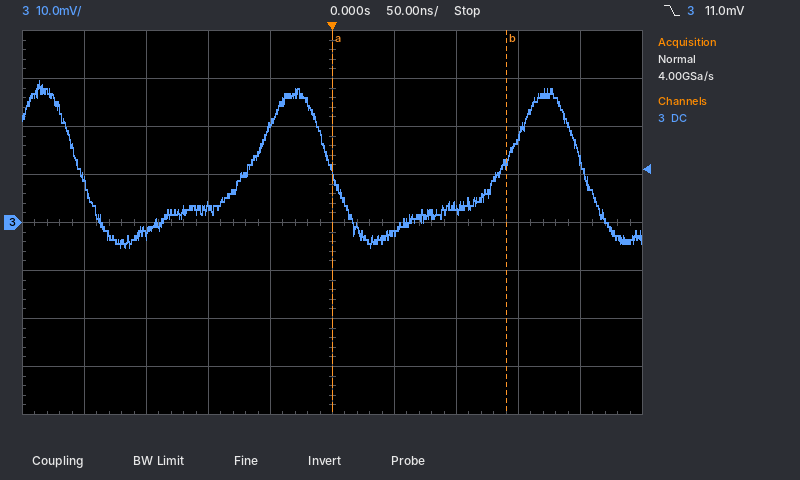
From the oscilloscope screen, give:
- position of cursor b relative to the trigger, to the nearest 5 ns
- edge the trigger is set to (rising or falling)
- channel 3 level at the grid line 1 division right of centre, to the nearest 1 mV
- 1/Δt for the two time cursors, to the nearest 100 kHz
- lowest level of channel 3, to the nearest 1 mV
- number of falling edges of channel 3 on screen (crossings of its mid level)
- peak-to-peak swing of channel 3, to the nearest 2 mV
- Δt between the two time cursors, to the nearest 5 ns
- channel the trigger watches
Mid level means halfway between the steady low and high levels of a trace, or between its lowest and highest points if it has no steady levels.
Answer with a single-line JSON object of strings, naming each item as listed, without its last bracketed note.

{"position of cursor b relative to the trigger, to the nearest 5 ns": "+140 ns", "edge the trigger is set to": "falling", "channel 3 level at the grid line 1 division right of centre, to the nearest 1 mV": "-2 mV", "1/Δt for the two time cursors, to the nearest 100 kHz": "7.1 MHz", "lowest level of channel 3, to the nearest 1 mV": "-5 mV", "number of falling edges of channel 3 on screen": "3", "peak-to-peak swing of channel 3, to the nearest 2 mV": "34 mV", "Δt between the two time cursors, to the nearest 5 ns": "140 ns", "channel the trigger watches": "channel 3"}
